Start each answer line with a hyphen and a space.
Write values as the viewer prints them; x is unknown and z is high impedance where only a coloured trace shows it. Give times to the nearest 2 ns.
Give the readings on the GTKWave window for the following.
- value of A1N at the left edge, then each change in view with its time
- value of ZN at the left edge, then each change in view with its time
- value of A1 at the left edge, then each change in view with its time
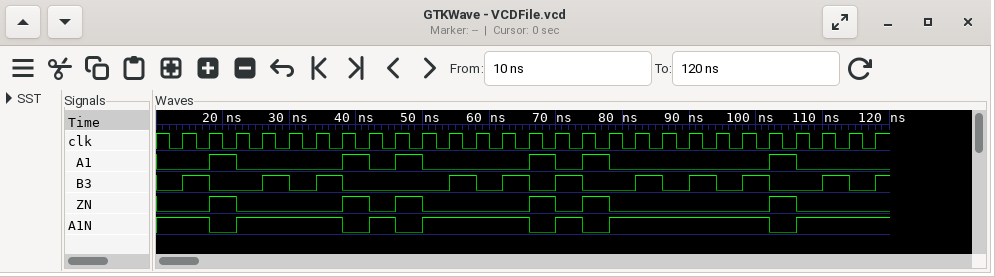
- 1, 0 at 18 ns, 1 at 22 ns, 0 at 38 ns, 1 at 42 ns, 0 at 46 ns, 1 at 50 ns, 0 at 66 ns, 1 at 70 ns, 0 at 74 ns, 1 at 78 ns, 0 at 102 ns, 1 at 106 ns
- 0, 1 at 18 ns, 0 at 22 ns, 1 at 38 ns, 0 at 42 ns, 1 at 46 ns, 0 at 50 ns, 1 at 66 ns, 0 at 70 ns, 1 at 74 ns, 0 at 78 ns, 1 at 102 ns, 0 at 106 ns
- 0, 1 at 18 ns, 0 at 22 ns, 1 at 38 ns, 0 at 42 ns, 1 at 46 ns, 0 at 50 ns, 1 at 66 ns, 0 at 70 ns, 1 at 74 ns, 0 at 78 ns, 1 at 102 ns, 0 at 106 ns
